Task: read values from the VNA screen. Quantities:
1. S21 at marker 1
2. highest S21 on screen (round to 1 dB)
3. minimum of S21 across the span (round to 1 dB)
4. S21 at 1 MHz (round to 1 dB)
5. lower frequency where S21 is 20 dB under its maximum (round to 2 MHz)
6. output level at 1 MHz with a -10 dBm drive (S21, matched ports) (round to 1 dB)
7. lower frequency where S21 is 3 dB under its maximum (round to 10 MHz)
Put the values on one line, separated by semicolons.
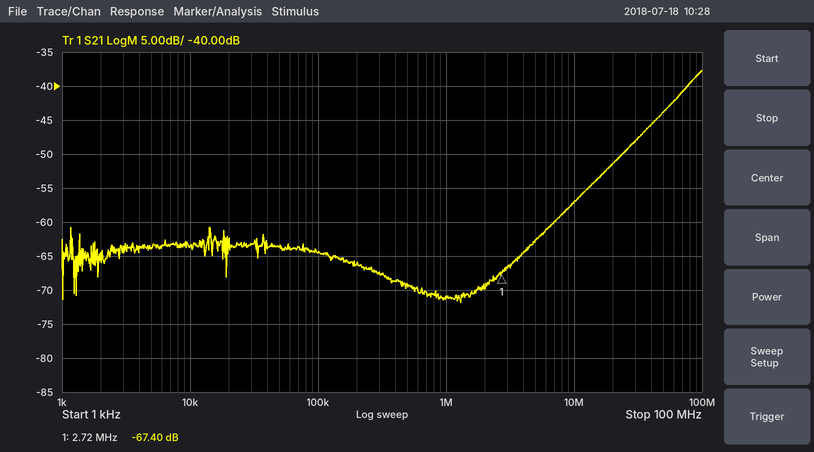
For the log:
-67.40 dB; -38 dB; -72 dB; -71 dB; 10 MHz; -81 dBm; 70 MHz
